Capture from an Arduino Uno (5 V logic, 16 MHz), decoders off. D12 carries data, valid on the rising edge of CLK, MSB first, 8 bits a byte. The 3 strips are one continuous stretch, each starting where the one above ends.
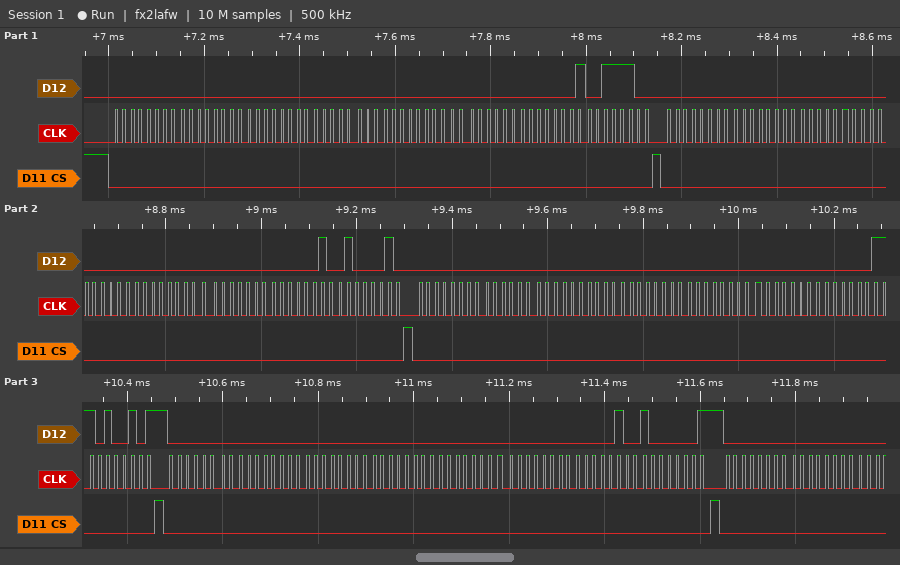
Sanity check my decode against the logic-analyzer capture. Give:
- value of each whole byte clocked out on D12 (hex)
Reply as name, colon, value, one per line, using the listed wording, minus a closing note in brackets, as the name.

value of each whole byte clocked out on D12: 00 00 00 00 00 00 01 3C 00 00 00 00 00 00 02 42 00 00 00 00 00 00 03 A5 00 00 00 00 00 00 04 81 00 00
